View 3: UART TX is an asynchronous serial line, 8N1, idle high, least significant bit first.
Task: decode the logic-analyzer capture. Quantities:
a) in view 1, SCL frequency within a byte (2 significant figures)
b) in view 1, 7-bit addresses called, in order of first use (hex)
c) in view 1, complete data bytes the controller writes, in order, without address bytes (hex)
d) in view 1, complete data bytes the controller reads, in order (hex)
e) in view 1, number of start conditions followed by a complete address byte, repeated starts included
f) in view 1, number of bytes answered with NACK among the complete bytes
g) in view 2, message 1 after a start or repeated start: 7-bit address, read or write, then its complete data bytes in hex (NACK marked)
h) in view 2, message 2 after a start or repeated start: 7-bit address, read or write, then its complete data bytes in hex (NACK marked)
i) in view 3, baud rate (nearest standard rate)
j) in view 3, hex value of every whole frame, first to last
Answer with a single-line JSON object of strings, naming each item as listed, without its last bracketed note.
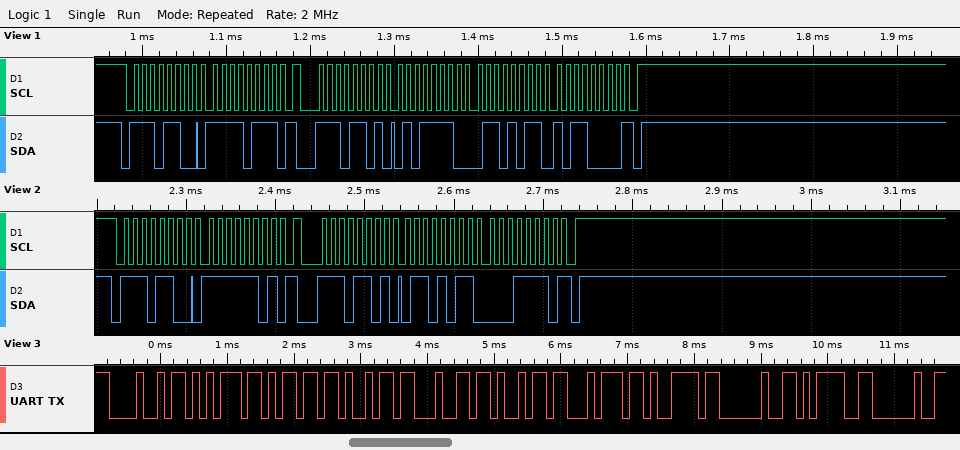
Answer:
{"in view 1, SCL frequency within a byte": "100 kHz", "in view 1, 7-bit addresses called, in order of first use": "0x76", "in view 1, complete data bytes the controller writes, in order, without address bytes": "F7", "in view 1, complete data bytes the controller reads, in order": "5E 6B B0", "in view 1, number of start conditions followed by a complete address byte, repeated starts included": "2", "in view 1, number of bytes answered with NACK among the complete bytes": "1", "in view 2, message 1 after a start or repeated start: 7-bit address, read or write, then its complete data bytes in hex": "0x76 write: FD", "in view 2, message 2 after a start or repeated start: 7-bit address, read or write, then its complete data bytes in hex": "0x76 read: 6B 1E NACK", "in view 3, baud rate": "9600 baud", "in view 3, hex value of every whole frame, first to last": "0x48 0x75 0x6D 0x69 0x64 0x69 0x74 0x79 0x20 0x3D 0x20"}
